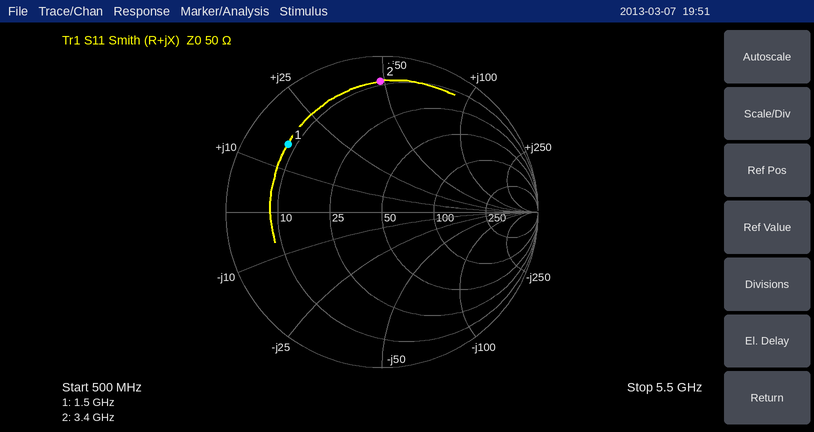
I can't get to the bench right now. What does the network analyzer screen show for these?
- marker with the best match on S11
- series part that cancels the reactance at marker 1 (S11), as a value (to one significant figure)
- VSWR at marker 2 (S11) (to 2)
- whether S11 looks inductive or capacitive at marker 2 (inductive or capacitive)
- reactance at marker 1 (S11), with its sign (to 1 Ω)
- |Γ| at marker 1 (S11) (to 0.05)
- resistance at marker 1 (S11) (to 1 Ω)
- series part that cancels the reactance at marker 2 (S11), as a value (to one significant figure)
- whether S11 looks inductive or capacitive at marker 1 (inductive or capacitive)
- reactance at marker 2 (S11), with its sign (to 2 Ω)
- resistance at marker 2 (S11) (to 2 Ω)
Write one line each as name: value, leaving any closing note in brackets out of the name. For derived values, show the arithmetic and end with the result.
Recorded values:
marker with the best match on S11: marker 1
series part that cancels the reactance at marker 1 (S11), as a value: C = 1/(2π × 1.5 GHz × 16 Ω) ≈ 7 pF
VSWR at marker 2 (S11): 12
whether S11 looks inductive or capacitive at marker 2: inductive
reactance at marker 1 (S11), with its sign: +16 Ω
|Γ| at marker 1 (S11): 0.75
resistance at marker 1 (S11): 8 Ω
series part that cancels the reactance at marker 2 (S11), as a value: C = 1/(2π × 3.4 GHz × 48 Ω) ≈ 1.0 pF
whether S11 looks inductive or capacitive at marker 1: inductive
reactance at marker 2 (S11), with its sign: +48 Ω
resistance at marker 2 (S11): 8 Ω
